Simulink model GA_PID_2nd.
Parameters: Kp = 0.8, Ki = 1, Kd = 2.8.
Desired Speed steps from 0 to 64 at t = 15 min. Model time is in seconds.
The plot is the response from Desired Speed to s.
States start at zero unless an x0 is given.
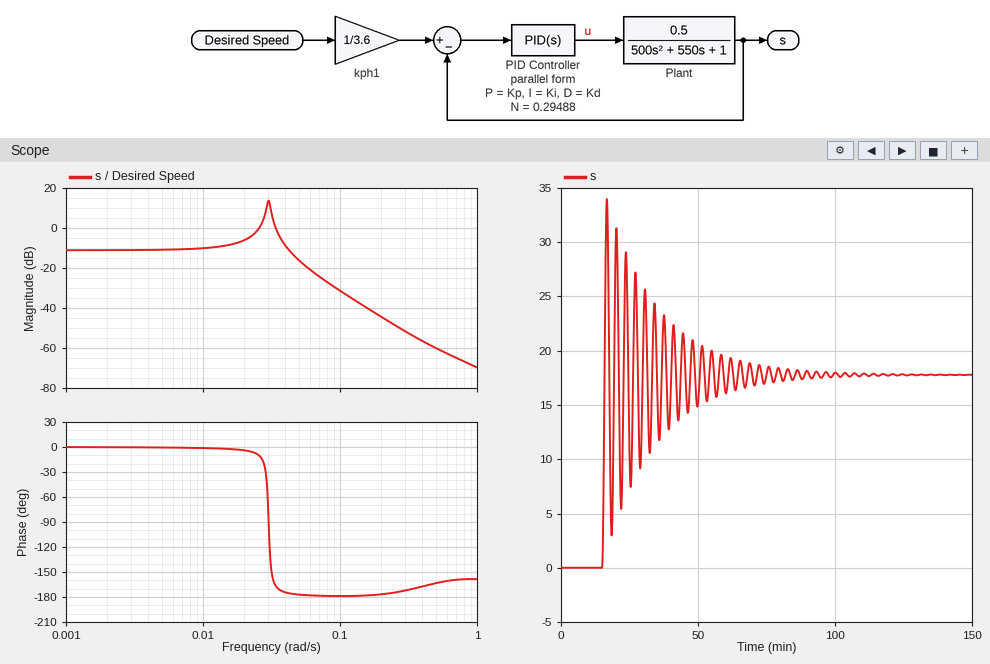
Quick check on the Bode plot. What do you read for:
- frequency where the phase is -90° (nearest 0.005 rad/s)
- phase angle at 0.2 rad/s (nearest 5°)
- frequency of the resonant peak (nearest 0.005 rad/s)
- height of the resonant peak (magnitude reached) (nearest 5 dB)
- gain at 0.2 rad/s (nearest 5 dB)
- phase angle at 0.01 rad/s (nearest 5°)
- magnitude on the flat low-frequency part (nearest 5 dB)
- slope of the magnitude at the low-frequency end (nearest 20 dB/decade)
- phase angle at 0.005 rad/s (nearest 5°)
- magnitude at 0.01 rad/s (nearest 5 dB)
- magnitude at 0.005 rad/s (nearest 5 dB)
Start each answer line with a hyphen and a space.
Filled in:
- 0.030 rad/s
- -175°
- 0.030 rad/s
- 15 dB
- -45 dB
- 0°
- -10 dB
- 0 dB/decade
- 0°
- -10 dB
- -10 dB
